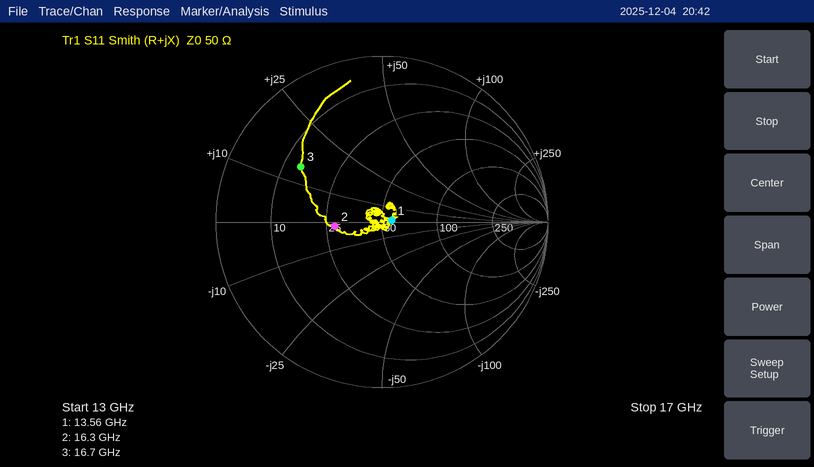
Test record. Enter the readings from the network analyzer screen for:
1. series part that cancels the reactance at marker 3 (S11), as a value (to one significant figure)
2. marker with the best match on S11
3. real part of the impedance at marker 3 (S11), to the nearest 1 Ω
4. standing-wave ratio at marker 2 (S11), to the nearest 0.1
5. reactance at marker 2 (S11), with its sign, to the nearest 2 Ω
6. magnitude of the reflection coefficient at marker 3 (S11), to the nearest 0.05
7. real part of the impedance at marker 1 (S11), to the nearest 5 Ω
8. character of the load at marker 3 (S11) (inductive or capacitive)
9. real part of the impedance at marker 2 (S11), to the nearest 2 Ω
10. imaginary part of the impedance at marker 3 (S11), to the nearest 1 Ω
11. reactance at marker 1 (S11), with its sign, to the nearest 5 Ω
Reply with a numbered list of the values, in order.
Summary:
1. 700 fF
2. marker 1
3. 14 Ω
4. 1.8
5. -2 Ω
6. 0.60
7. 55 Ω
8. inductive
9. 28 Ω
10. +14 Ω
11. 0 Ω
